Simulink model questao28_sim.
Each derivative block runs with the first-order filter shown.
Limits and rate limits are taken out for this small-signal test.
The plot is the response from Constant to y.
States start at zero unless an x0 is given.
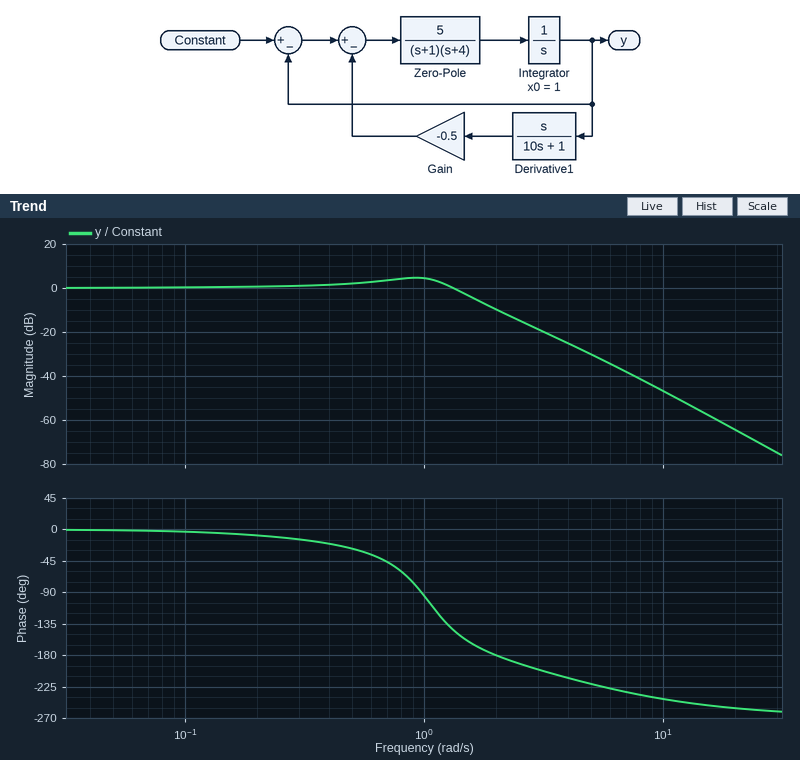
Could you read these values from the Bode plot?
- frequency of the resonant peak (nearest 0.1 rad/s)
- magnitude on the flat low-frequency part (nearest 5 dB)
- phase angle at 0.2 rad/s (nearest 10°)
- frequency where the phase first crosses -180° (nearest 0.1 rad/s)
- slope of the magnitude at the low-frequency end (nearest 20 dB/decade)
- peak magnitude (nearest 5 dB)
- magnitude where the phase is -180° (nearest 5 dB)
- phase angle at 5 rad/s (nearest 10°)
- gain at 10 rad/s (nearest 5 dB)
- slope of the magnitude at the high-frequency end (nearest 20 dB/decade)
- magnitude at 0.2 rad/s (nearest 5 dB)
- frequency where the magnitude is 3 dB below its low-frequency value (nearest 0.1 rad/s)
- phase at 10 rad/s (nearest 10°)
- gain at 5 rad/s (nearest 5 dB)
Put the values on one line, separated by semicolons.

0.9 rad/s; 0 dB; -10°; 2.0 rad/s; 0 dB/decade; 5 dB; -10 dB; -220°; -45 dB; -60 dB/decade; 0 dB; 1.5 rad/s; -240°; -30 dB
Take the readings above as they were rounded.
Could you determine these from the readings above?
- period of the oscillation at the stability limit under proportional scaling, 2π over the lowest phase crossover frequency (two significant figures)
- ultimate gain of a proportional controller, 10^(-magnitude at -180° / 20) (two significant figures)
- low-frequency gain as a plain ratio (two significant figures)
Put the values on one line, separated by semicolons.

3.1 s; 3.2; 1.0
